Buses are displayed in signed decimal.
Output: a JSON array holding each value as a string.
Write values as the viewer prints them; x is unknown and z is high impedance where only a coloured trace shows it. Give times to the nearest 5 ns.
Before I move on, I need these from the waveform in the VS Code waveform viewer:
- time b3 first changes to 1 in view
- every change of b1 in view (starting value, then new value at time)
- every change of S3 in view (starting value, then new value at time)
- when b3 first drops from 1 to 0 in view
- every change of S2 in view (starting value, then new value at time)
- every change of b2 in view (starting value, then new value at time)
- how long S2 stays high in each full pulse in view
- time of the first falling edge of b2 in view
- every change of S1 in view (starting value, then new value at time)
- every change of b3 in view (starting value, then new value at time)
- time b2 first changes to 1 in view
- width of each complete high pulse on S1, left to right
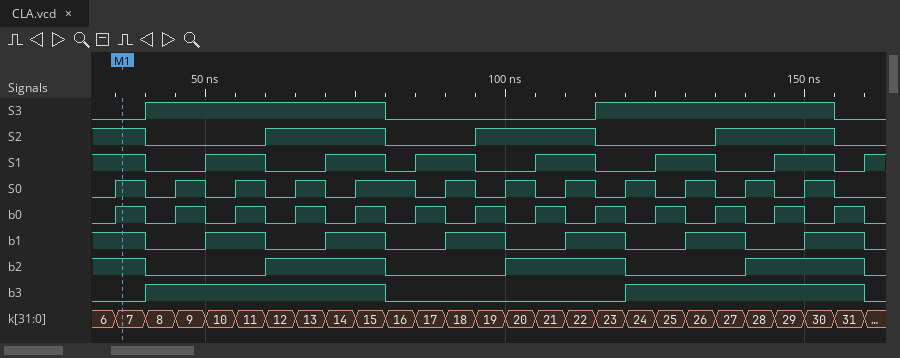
["40 ns", "1, 0 at 40 ns, 1 at 50 ns, 0 at 60 ns, 1 at 70 ns, 0 at 80 ns, 1 at 90 ns, 0 at 100 ns, 1 at 110 ns, 0 at 120 ns, 1 at 130 ns, 0 at 140 ns, 1 at 150 ns, 0 at 160 ns", "0, 1 at 40 ns, 0 at 80 ns, 1 at 115 ns, 0 at 155 ns", "80 ns", "1, 0 at 40 ns, 1 at 60 ns, 0 at 80 ns, 1 at 95 ns, 0 at 115 ns, 1 at 135 ns, 0 at 155 ns", "1, 0 at 40 ns, 1 at 60 ns, 0 at 80 ns, 1 at 100 ns, 0 at 120 ns, 1 at 140 ns, 0 at 160 ns", "20 ns, 20 ns, 20 ns", "40 ns", "1, 0 at 40 ns, 1 at 50 ns, 0 at 60 ns, 1 at 70 ns, 0 at 80 ns, 1 at 85 ns, 0 at 95 ns, 1 at 105 ns, 0 at 115 ns, 1 at 125 ns, 0 at 135 ns, 1 at 145 ns, 0 at 155 ns, 1 at 160 ns", "0, 1 at 40 ns, 0 at 80 ns, 1 at 120 ns, 0 at 160 ns", "60 ns", "10 ns, 10 ns, 10 ns, 10 ns, 10 ns, 10 ns"]
